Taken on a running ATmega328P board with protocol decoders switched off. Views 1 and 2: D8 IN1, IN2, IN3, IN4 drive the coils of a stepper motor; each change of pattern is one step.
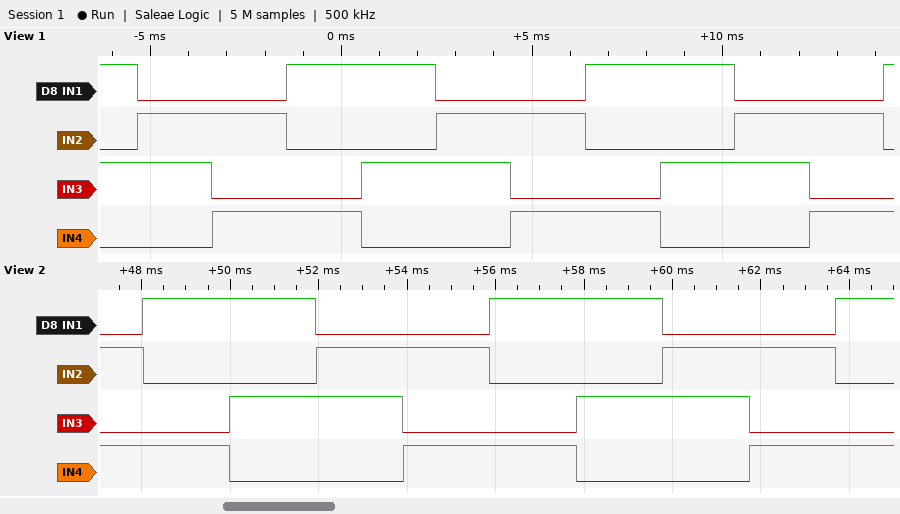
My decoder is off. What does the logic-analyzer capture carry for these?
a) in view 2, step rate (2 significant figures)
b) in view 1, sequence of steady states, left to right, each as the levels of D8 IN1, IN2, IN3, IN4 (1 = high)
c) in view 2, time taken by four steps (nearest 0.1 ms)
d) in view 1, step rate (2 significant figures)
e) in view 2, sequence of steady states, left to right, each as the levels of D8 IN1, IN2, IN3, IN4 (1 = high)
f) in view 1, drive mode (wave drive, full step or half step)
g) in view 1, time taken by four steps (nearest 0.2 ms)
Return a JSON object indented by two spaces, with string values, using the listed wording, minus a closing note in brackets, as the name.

{
  "in view 2, step rate": "510 steps/s",
  "in view 1, sequence of steady states, left to right, each as the levels of D8 IN1, IN2, IN3, IN4": "1010 0110 0101 1001 1010 0110 0101 1001 1010 0110 0101 1001",
  "in view 2, time taken by four steps": "7.8 ms",
  "in view 1, step rate": "510 steps/s",
  "in view 2, sequence of steady states, left to right, each as the levels of D8 IN1, IN2, IN3, IN4": "0101 1001 1010 0110 0101 1001 1010 0110 0101 1001",
  "in view 1, drive mode": "full step",
  "in view 1, time taken by four steps": "7.8 ms"
}
